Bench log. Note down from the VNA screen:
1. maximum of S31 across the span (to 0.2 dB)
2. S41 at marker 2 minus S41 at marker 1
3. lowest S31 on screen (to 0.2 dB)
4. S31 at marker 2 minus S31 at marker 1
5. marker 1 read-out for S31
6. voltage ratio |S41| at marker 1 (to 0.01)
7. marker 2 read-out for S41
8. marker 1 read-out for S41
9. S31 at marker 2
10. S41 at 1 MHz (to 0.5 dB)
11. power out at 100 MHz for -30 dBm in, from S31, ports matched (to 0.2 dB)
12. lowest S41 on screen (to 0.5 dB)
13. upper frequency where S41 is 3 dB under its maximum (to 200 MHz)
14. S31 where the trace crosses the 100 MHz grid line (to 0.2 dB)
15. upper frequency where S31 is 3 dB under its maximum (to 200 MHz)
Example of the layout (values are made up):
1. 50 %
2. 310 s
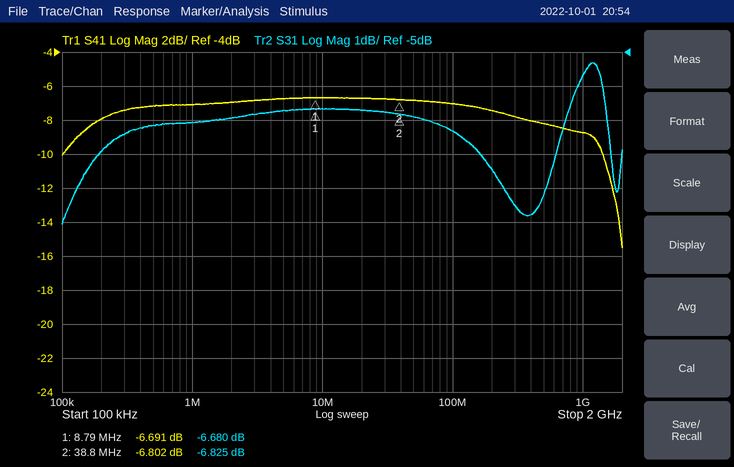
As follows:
1. -5.4 dB
2. -0.111 dB
3. -10.0 dB
4. -0.145 dB
5. -6.680 dB
6. 0.46
7. -6.802 dB
8. -6.691 dB
9. -6.825 dB
10. -7.0 dB
11. -37.4 dBm
12. -15.5 dB
13. 1.4 GHz
14. -7.4 dB
15. 1.6 GHz
